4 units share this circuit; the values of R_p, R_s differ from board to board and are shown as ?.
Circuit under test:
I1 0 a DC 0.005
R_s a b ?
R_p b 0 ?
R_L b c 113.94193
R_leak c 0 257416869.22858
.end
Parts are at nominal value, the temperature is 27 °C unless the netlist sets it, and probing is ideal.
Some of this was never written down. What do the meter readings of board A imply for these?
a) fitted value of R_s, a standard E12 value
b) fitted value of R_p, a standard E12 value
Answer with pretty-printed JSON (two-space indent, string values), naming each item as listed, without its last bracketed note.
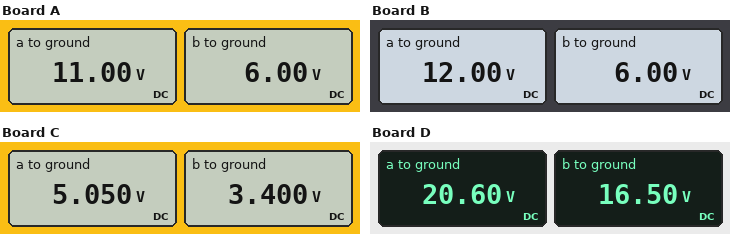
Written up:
{
  "fitted value of R_s, a standard E12 value": "1 kΩ",
  "fitted value of R_p, a standard E12 value": "1.2 kΩ"
}
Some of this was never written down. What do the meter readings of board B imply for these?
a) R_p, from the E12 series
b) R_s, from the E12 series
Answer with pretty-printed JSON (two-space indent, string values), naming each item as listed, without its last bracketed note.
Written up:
{
  "R_p, from the E12 series": "1.2 kΩ",
  "R_s, from the E12 series": "1.2 kΩ"
}
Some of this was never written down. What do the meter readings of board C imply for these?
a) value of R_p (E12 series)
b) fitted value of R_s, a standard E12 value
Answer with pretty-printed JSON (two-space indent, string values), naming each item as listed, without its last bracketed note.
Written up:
{
  "value of R_p": "680 Ω",
  "fitted value of R_s, a standard E12 value": "330 Ω"
}
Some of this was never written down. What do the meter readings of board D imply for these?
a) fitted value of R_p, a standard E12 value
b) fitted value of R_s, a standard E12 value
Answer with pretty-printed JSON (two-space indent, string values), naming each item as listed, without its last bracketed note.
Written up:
{
  "fitted value of R_p, a standard E12 value": "3.3 kΩ",
  "fitted value of R_s, a standard E12 value": "820 Ω"
}
